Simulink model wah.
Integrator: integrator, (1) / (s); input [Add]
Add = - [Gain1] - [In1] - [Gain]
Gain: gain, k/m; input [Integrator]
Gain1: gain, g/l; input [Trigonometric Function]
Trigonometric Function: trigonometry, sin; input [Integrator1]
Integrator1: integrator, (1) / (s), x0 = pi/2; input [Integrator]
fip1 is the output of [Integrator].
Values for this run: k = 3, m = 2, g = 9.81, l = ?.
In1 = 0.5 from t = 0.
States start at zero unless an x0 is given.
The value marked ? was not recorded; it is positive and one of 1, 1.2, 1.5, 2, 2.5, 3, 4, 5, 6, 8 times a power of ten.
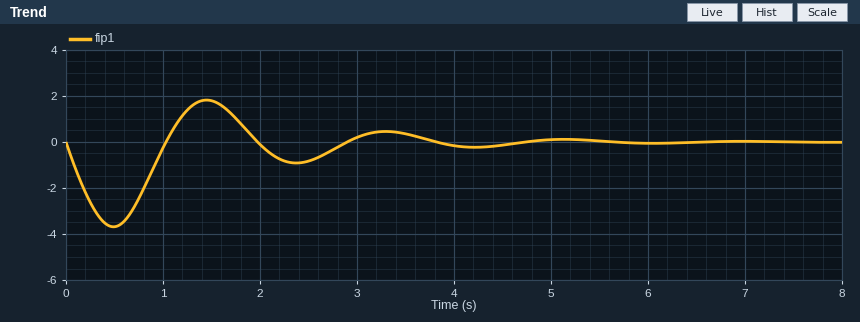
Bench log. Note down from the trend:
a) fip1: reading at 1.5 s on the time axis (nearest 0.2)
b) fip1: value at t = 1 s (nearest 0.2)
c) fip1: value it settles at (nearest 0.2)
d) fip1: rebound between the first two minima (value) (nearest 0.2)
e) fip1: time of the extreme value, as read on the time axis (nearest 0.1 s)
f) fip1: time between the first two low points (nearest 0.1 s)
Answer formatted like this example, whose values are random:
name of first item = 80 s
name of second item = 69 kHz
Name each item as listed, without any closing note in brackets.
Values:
fip1: reading at 1.5 s on the time axis = 1.8
fip1: value at t = 1 s = -0.2
fip1: value it settles at = 0.0
fip1: rebound between the first two minima (value) = 1.8
fip1: time of the extreme value, as read on the time axis = 0.5 s
fip1: time between the first two low points = 1.9 s
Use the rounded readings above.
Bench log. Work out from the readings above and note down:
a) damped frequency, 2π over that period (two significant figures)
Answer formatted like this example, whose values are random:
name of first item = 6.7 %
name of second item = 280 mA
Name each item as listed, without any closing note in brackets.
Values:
damped frequency, 2π over that period = 3.3 rad/s
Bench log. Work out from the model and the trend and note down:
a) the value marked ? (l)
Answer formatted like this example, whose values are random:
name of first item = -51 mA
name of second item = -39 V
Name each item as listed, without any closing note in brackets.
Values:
the value marked ? = 0.8
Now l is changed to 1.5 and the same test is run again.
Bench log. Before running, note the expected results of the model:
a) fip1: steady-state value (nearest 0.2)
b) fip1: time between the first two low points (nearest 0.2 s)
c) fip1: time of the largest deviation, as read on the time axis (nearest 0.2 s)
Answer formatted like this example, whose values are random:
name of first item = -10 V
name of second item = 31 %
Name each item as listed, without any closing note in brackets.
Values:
fip1: steady-state value = 0.0
fip1: time between the first two low points = 2.6 s
fip1: time of the largest deviation, as read on the time axis = 0.6 s
